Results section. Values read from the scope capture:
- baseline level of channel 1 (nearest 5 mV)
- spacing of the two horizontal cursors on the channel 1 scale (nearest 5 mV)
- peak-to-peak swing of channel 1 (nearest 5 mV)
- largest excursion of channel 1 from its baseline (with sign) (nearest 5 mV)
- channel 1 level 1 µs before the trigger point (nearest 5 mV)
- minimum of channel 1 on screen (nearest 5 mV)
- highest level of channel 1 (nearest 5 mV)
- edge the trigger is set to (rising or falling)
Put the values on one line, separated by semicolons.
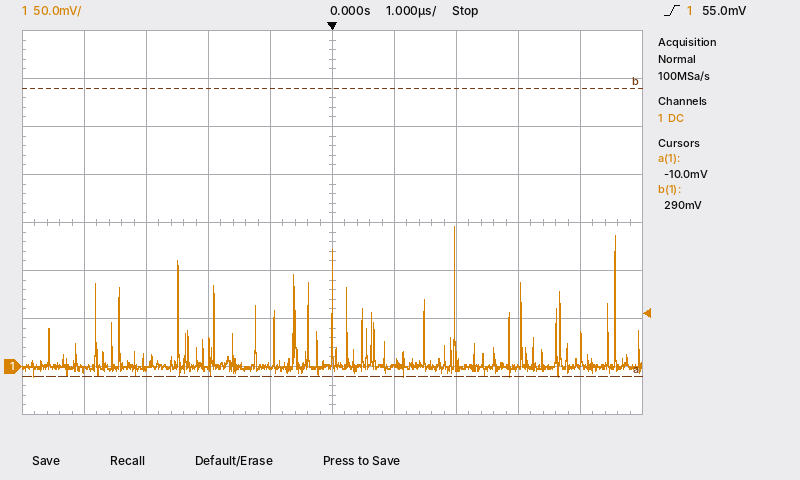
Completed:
0 mV; 300 mV; 155 mV; +145 mV; 0 mV; -10 mV; 145 mV; rising
